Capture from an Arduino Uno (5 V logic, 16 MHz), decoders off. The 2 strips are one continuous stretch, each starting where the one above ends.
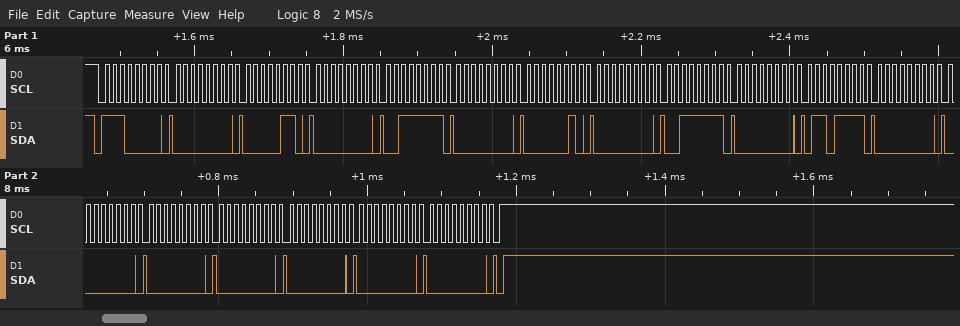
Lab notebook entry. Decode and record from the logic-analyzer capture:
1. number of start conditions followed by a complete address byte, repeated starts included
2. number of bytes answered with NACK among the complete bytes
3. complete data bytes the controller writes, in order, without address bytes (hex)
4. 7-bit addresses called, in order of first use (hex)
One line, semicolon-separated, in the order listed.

1; 0; 00 06 00 3F 00 02 00 3F 00 6F 00 00 00 00 00 00 00; 0x70
